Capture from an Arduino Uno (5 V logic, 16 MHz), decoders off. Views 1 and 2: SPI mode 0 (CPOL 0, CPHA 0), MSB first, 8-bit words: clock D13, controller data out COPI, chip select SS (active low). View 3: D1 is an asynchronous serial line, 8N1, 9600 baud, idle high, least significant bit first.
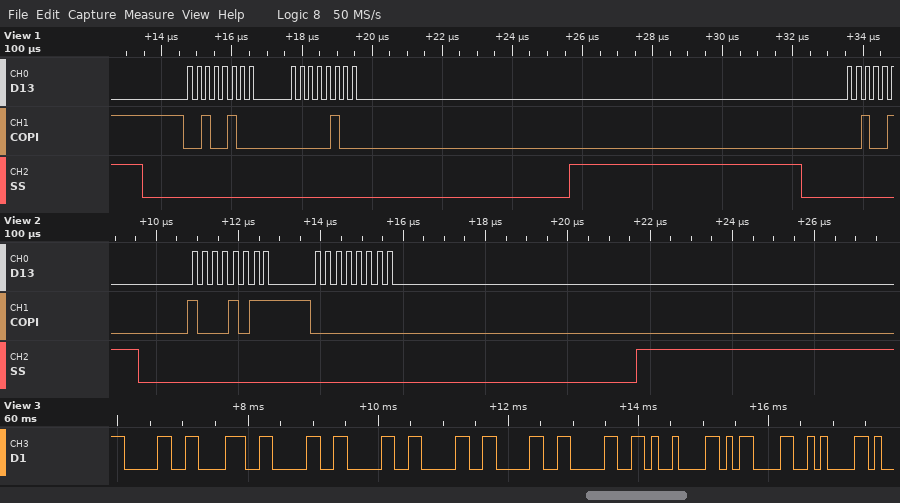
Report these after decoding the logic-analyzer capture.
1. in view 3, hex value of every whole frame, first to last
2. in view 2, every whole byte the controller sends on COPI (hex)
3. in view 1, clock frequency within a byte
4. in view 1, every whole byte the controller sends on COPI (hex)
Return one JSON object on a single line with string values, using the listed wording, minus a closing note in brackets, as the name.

{"in view 3, hex value of every whole frame, first to last": "30 38 30 30 30 30 30 09 0D 0A", "in view 2, every whole byte the controller sends on COPI": "8B 00", "in view 1, clock frequency within a byte": "4 MHz", "in view 1, every whole byte the controller sends on COPI": "24 04"}
